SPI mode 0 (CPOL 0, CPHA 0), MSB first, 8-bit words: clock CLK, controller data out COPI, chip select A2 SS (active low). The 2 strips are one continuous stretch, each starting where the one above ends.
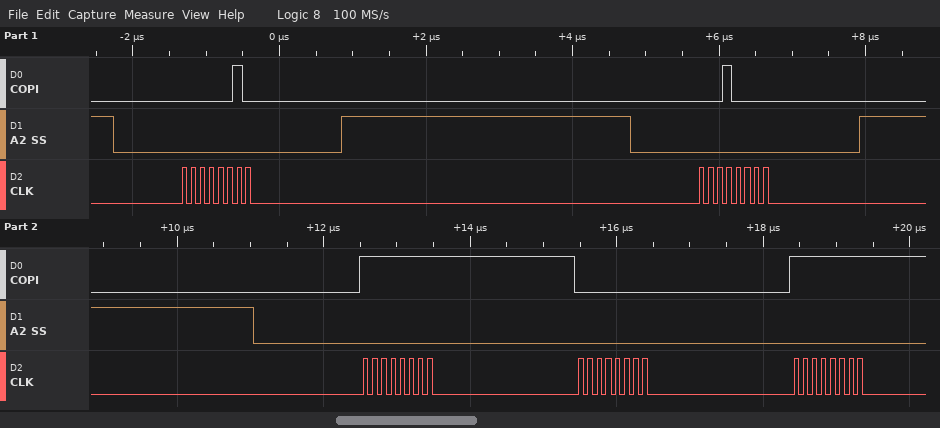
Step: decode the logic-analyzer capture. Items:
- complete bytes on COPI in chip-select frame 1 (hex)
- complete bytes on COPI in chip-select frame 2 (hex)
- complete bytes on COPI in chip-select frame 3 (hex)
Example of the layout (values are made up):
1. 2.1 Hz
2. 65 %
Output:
1. 02
2. 10
3. FF 00 FF
